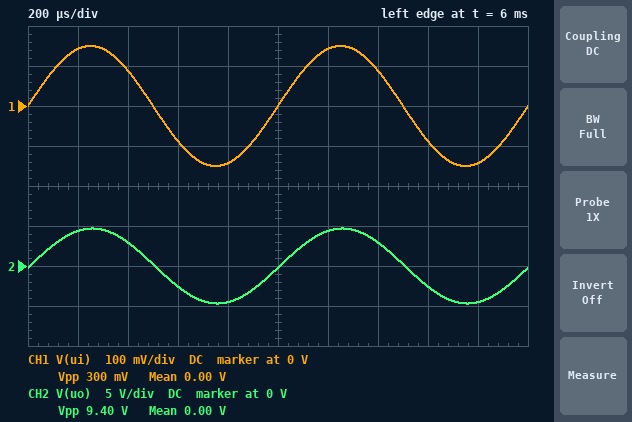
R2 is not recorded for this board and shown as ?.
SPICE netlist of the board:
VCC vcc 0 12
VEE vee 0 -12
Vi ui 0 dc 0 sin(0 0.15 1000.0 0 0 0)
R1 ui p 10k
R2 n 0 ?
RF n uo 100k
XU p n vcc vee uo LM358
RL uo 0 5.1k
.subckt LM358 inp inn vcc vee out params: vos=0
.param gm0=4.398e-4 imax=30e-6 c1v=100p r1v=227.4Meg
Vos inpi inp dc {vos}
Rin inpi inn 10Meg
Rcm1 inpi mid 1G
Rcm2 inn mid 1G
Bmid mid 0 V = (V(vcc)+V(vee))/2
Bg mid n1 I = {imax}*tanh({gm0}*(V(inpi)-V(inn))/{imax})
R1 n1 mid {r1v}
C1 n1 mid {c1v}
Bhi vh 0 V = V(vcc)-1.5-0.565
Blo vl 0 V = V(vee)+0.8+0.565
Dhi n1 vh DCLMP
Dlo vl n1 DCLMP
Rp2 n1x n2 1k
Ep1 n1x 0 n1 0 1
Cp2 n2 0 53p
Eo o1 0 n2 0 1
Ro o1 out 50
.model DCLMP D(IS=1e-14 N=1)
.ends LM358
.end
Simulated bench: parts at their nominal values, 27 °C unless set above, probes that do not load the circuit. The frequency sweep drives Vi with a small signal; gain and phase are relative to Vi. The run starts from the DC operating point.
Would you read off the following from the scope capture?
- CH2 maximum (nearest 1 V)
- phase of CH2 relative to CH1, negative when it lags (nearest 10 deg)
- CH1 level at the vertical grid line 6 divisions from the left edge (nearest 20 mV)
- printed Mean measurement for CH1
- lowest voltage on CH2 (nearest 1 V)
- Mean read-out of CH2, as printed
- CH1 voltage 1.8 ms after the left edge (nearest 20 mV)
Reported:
5 V
0 deg
140 mV
0.00 V
-5 V
0.00 V
-140 mV
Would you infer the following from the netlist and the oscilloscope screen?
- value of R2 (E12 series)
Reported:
3.3 kΩ
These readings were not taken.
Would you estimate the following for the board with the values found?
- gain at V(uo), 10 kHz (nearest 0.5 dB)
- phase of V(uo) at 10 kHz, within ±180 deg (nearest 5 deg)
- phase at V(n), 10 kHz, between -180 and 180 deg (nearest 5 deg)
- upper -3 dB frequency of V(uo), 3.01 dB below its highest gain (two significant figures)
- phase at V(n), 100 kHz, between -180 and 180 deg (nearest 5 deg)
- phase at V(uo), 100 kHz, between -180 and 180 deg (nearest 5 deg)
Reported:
29.0 dB
-25 deg
-25 deg
22 kHz
-80 deg
-80 deg
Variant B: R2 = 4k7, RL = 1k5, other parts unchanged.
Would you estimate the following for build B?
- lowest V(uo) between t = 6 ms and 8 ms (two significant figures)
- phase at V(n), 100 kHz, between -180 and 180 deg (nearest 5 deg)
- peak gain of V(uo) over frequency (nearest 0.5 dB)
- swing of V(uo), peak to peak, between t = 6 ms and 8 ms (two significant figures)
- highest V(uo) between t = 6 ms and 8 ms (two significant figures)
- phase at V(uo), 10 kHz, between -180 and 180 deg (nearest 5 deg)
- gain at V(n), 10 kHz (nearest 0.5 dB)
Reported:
-3.3 V
-75 deg
27.0 dB
6.7 V
3.3 V
-20 deg
-0.5 dB
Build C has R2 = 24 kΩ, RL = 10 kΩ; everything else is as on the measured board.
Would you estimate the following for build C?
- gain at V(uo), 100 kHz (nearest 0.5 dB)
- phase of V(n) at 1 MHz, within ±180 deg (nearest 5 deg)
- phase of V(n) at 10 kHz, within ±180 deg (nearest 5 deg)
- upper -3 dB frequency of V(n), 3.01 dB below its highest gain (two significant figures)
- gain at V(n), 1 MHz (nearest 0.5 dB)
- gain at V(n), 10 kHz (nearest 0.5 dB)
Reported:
12.5 dB
-100 deg
-5 deg
140 kHz
-17.5 dB
0 dB
